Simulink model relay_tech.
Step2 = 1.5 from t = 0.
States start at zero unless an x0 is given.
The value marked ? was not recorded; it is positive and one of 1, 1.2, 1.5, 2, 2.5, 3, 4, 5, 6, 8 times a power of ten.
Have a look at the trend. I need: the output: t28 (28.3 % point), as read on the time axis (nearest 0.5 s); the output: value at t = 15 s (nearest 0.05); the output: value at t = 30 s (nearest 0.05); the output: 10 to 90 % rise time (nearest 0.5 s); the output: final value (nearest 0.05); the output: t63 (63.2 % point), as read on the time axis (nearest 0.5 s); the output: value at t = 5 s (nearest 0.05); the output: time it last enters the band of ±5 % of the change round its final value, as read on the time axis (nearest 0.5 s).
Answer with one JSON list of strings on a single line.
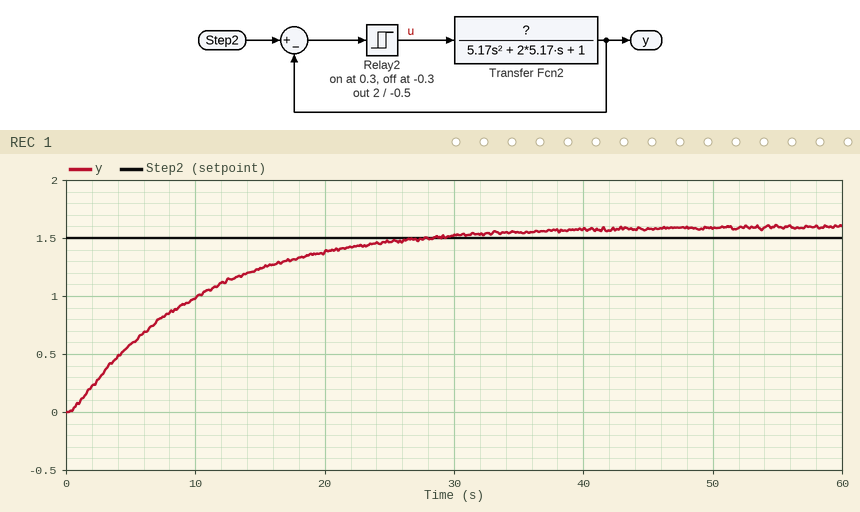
["4.0 s", "1.25", "1.50", "21.5 s", "1.60", "10.5 s", "0.60", "30.0 s"]
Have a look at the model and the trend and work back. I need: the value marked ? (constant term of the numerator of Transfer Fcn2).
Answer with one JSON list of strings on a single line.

["0.8"]
